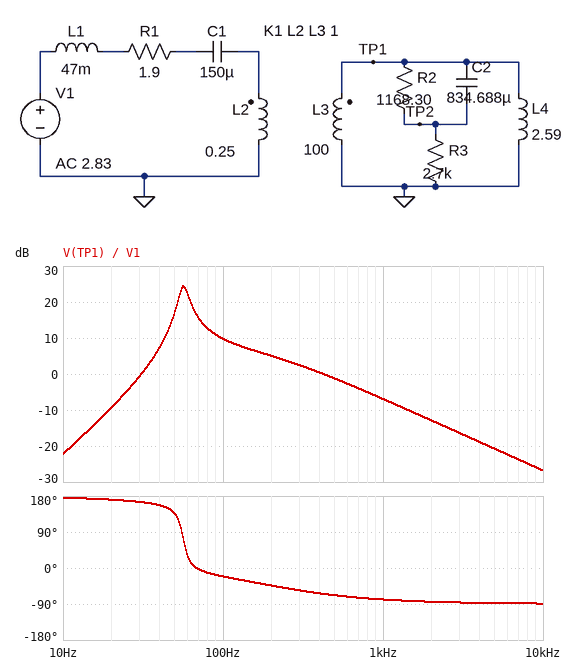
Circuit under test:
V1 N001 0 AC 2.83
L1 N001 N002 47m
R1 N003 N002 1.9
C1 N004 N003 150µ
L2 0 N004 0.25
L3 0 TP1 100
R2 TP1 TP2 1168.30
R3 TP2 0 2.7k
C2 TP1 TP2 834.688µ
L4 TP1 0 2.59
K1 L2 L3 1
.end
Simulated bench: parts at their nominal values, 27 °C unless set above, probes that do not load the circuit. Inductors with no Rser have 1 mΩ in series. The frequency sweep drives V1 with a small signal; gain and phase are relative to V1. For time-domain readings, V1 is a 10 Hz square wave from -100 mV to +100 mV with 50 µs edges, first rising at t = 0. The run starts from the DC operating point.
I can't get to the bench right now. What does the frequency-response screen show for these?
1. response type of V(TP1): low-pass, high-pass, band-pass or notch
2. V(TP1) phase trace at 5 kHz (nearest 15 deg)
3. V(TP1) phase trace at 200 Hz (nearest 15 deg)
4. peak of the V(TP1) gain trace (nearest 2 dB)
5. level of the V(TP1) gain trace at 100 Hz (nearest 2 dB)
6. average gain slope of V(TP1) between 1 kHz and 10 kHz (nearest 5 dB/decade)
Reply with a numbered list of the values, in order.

1. band-pass
2. -90 deg
3. -45 deg
4. 24 dB
5. 10 dB
6. -20 dB/decade
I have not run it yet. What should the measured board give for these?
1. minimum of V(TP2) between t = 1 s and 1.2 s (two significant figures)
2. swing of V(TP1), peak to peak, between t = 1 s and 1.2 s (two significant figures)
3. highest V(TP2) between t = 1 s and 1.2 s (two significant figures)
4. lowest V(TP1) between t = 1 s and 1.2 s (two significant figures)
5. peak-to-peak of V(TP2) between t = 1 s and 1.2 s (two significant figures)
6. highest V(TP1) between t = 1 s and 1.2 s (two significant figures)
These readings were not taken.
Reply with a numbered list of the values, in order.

1. -330 mV
2. 660 mV
3. 330 mV
4. -330 mV
5. 660 mV
6. 330 mV
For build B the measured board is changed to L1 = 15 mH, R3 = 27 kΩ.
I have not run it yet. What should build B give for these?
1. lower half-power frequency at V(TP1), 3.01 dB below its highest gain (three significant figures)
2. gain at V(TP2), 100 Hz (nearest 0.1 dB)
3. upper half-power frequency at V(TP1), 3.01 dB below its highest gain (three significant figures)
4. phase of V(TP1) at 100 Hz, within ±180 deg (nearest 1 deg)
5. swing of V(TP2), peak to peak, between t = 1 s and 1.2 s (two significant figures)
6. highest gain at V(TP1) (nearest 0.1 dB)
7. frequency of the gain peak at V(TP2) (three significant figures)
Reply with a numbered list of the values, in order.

1. 82.6 Hz
2. 27.1 dB
3. 98.8 Hz
4. 34 deg
5. 2.5 V
6. 30.6 dB
7. 89.6 Hz
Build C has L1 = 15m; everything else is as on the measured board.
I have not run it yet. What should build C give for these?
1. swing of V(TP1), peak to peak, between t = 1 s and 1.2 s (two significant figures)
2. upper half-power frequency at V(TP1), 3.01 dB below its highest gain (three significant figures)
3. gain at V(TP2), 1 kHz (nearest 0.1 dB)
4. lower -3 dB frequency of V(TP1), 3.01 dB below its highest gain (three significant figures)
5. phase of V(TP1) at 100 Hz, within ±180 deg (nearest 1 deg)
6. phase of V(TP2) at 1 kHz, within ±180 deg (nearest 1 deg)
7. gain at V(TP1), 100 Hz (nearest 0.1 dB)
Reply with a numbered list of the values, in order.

1. 1.6 V
2. 111 Hz
3. 3.0 dB
4. 80.4 Hz
5. 34 deg
6. -75 deg
7. 24.6 dB
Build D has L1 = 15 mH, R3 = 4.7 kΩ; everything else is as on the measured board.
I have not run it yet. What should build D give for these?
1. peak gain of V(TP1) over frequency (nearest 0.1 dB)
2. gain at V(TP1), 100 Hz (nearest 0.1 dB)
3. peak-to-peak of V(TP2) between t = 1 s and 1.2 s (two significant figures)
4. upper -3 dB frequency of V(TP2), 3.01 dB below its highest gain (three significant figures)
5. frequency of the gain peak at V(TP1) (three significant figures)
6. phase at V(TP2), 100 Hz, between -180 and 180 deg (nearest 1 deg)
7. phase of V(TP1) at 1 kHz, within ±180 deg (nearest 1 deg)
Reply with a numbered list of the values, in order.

1. 27.5 dB
2. 25.7 dB
3. 1.9 V
4. 105 Hz
5. 90.6 Hz
6. 34 deg
7. -66 deg
